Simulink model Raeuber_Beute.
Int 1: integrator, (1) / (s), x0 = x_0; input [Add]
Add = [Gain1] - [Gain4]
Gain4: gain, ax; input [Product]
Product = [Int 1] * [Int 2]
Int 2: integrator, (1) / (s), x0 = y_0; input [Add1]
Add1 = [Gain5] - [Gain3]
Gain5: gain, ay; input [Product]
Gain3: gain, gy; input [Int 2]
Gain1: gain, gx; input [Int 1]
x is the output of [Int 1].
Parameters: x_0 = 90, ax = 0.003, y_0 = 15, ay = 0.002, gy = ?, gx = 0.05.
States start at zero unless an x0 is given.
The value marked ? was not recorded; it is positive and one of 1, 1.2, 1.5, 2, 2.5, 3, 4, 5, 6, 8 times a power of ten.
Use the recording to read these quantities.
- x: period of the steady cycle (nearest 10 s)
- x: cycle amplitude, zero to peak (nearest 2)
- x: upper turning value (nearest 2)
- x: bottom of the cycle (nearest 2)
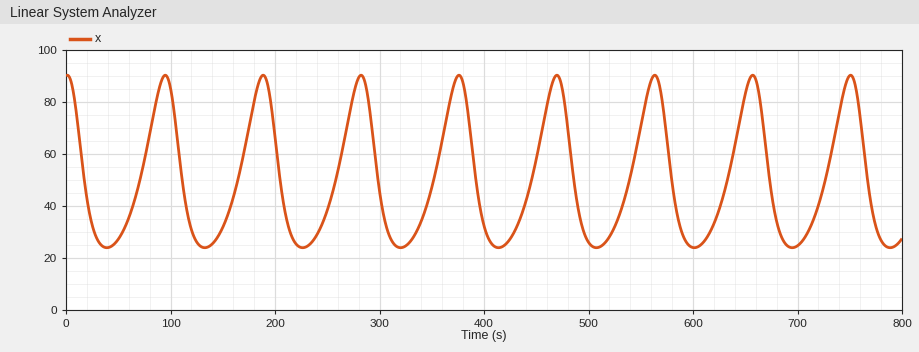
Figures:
90 s
34
90
24
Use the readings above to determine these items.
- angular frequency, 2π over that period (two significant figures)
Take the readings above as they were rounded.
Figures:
0.070 rad/s
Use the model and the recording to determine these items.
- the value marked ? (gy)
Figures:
0.1
